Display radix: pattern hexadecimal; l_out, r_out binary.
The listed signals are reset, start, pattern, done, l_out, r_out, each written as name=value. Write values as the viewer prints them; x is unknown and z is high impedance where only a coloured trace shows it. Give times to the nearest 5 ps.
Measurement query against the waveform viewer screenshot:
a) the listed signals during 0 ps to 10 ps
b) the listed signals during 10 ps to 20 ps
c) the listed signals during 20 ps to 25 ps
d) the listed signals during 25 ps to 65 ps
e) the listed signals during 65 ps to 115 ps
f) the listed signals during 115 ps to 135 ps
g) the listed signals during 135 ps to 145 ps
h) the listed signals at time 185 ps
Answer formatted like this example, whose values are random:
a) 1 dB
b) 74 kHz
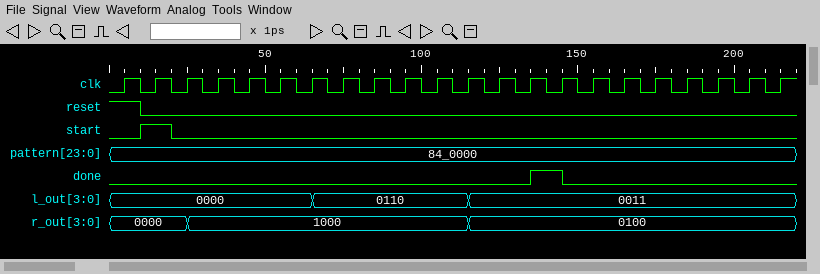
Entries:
a) reset=1, start=0, pattern=84_0000, done=0, l_out=0000, r_out=0000
b) reset=0, start=1, pattern=84_0000, done=0, l_out=0000, r_out=0000
c) reset=0, start=0, pattern=84_0000, done=0, l_out=0000, r_out=0000
d) reset=0, start=0, pattern=84_0000, done=0, l_out=0000, r_out=1000
e) reset=0, start=0, pattern=84_0000, done=0, l_out=0110, r_out=1000
f) reset=0, start=0, pattern=84_0000, done=0, l_out=0011, r_out=0100
g) reset=0, start=0, pattern=84_0000, done=1, l_out=0011, r_out=0100
h) reset=0, start=0, pattern=84_0000, done=0, l_out=0011, r_out=0100
